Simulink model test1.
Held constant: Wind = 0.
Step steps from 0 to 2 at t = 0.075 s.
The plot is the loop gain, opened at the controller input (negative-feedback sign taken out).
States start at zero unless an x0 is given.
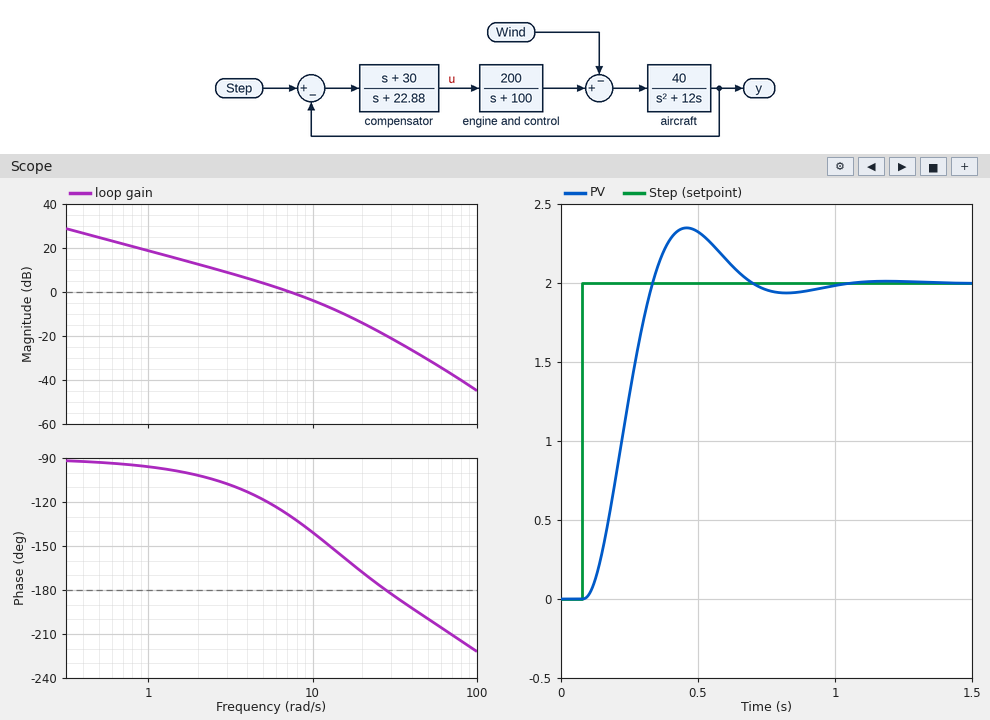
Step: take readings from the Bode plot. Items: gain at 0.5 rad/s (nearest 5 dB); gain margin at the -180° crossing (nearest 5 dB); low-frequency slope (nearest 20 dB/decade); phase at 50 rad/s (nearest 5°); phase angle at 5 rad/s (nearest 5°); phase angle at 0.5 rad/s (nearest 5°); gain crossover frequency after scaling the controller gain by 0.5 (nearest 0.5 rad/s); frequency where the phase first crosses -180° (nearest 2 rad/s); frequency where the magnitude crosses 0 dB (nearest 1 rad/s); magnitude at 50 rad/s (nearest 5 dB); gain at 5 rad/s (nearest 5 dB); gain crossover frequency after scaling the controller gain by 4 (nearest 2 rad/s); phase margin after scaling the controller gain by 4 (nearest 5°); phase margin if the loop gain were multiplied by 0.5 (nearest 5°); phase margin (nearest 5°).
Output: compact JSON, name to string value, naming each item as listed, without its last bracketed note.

{"gain at 0.5 rad/s": "25 dB", "gain margin at the -180° crossing": "20 dB", "low-frequency slope": "-20 dB/decade", "phase at 50 rad/s": "-200°", "phase angle at 5 rad/s": "-120°", "phase angle at 0.5 rad/s": "-95°", "gain crossover frequency after scaling the controller gain by 0.5": "4.0 rad/s", "frequency where the phase first crosses -180°": "28 rad/s", "frequency where the magnitude crosses 0 dB": "7 rad/s", "magnitude at 50 rad/s": "-30 dB", "gain at 5 rad/s": "5 dB", "gain crossover frequency after scaling the controller gain by 4": "18 rad/s", "phase margin after scaling the controller gain by 4": "15°", "phase margin if the loop gain were multiplied by 0.5": "65°", "phase margin": "50°"}
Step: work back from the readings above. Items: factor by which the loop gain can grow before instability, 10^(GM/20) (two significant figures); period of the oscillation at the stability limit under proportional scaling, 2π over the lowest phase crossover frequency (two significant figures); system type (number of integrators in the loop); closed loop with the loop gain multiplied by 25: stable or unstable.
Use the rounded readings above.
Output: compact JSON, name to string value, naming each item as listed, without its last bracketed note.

{"factor by which the loop gain can grow before instability, 10^(GM/20)": "10", "period of the oscillation at the stability limit under proportional scaling, 2π over the lowest phase crossover frequency": "0.22 s", "system type": "1", "closed loop with the loop gain multiplied by 25: stable or unstable": "unstable"}
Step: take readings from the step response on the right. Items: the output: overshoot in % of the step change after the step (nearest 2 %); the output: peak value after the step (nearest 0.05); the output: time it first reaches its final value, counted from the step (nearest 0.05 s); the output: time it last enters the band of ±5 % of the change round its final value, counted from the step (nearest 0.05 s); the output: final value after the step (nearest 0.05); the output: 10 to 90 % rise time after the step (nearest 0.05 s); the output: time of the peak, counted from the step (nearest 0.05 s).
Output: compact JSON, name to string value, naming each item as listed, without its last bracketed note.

{"the output: overshoot in % of the step change after the step": "18 %", "the output: peak value after the step": "2.35", "the output: time it first reaches its final value, counted from the step": "0.25 s", "the output: time it last enters the band of ±5 % of the change round its final value, counted from the step": "0.55 s", "the output: final value after the step": "2.00", "the output: 10 to 90 % rise time after the step": "0.15 s", "the output: time of the peak, counted from the step": "0.40 s"}
